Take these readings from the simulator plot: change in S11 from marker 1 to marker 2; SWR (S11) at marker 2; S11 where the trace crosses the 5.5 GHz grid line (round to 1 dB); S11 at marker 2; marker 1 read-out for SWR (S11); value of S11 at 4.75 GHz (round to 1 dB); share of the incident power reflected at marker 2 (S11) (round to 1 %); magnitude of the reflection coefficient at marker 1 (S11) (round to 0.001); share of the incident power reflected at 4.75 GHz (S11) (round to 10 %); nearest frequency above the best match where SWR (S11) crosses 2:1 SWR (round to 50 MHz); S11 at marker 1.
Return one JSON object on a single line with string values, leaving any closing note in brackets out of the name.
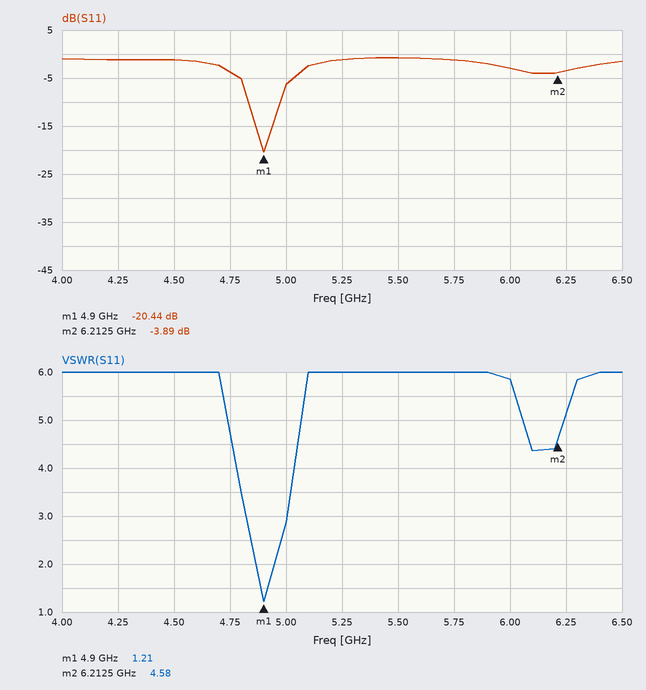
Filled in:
{"change in S11 from marker 1 to marker 2": "16.55 dB", "SWR (S11) at marker 2": "4.58", "S11 where the trace crosses the 5.5 GHz grid line": "-1 dB", "S11 at marker 2": "-3.89 dB", "marker 1 read-out for SWR": "1.21", "value of S11 at 4.75 GHz": "-4 dB", "share of the incident power reflected at marker 2 (S11)": "41 %", "magnitude of the reflection coefficient at marker 1 (S11)": "0.095", "share of the incident power reflected at 4.75 GHz (S11)": "40 %", "nearest frequency above the best match where SWR (S11) crosses 2:1 SWR": "4.95 GHz", "S11 at marker 1": "-20.44 dB"}
